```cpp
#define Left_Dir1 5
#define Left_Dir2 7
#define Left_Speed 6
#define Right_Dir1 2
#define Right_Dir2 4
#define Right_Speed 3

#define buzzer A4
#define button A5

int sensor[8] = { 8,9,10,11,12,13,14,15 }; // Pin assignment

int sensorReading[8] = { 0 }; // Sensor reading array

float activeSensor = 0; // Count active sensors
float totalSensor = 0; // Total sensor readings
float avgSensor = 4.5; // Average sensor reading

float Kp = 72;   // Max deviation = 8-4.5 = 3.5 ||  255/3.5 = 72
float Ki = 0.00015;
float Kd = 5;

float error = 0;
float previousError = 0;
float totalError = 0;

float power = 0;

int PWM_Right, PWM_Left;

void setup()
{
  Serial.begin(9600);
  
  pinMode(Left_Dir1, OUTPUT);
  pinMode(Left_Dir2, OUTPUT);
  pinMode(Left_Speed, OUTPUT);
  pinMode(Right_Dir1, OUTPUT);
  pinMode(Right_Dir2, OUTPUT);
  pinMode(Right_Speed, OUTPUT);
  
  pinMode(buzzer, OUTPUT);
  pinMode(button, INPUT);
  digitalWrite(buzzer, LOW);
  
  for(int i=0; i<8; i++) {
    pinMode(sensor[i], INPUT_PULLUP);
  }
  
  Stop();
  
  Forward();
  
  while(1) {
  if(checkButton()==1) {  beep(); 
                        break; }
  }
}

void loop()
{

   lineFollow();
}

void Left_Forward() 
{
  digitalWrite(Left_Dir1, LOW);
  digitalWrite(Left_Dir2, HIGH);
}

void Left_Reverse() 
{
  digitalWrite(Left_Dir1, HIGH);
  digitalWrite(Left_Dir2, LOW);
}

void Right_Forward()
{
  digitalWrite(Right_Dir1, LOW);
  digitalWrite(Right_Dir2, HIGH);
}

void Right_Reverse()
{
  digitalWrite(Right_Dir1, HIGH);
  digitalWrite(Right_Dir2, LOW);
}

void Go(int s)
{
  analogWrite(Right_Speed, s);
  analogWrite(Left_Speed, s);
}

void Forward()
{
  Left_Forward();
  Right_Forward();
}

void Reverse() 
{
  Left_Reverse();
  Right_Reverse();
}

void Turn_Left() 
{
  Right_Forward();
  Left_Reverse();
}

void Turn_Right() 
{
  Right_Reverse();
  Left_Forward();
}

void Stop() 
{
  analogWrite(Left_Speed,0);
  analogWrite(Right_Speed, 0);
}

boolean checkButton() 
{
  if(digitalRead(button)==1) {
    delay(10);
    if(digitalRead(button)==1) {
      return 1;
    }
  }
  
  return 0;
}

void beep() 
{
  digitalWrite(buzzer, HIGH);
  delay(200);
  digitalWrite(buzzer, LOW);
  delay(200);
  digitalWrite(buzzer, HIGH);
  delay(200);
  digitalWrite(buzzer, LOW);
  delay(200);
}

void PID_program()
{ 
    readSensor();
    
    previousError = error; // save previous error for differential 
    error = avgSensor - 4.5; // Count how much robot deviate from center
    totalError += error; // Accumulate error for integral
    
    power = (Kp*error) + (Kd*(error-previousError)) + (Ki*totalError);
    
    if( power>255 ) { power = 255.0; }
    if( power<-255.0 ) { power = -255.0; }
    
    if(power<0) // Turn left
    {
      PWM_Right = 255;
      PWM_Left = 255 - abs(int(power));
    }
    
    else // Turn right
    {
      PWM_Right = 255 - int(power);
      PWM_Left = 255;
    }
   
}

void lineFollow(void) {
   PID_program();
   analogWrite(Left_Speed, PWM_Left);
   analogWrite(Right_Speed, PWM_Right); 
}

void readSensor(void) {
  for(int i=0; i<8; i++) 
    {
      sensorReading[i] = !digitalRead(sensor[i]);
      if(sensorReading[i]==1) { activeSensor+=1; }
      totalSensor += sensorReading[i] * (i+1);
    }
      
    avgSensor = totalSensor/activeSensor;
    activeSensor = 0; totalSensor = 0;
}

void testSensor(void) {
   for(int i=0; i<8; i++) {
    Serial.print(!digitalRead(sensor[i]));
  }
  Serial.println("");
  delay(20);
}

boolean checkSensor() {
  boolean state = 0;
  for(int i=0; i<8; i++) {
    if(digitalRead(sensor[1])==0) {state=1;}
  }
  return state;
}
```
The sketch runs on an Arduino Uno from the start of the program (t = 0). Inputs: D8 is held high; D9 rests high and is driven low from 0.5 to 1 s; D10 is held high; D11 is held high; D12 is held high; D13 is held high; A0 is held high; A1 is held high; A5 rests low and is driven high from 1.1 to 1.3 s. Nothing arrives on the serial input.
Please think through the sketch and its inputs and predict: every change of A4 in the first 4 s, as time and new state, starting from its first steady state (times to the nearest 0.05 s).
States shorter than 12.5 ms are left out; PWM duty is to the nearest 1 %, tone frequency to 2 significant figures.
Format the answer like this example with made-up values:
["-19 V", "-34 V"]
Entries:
["0 s low; 1.1 s high; 1.3 s low; 1.5 s high; 1.7 s low"]
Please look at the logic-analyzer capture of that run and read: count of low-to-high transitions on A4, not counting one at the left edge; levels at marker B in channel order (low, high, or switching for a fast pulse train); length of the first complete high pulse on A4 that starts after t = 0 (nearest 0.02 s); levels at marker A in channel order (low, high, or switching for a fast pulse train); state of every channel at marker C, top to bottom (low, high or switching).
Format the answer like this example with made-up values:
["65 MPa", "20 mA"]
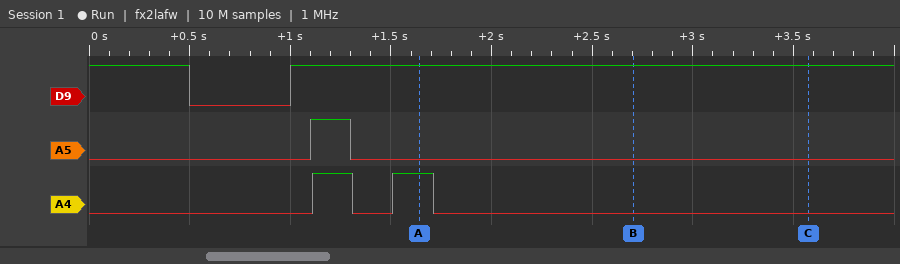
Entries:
["2", "D9 high, A5 low, A4 low", "0.20 s", "D9 high, A5 low, A4 high", "D9 high, A5 low, A4 low"]
